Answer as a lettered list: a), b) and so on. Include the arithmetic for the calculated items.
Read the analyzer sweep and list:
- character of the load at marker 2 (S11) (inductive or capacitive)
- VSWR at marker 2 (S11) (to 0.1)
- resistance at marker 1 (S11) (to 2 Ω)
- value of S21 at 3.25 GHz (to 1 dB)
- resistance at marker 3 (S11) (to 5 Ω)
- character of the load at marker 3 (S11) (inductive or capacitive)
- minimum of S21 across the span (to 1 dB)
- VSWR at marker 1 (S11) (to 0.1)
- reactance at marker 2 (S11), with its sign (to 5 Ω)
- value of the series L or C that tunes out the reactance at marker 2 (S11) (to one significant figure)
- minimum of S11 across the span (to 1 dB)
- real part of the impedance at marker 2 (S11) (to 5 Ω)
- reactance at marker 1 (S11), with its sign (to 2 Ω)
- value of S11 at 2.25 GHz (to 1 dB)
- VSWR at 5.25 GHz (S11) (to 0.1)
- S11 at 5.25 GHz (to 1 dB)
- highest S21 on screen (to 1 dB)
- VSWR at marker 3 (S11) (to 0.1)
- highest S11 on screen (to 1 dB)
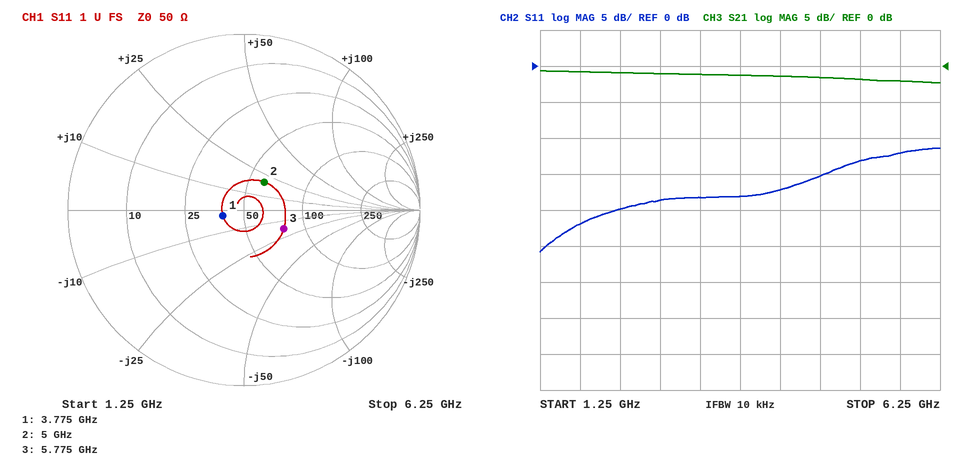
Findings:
a) inductive
b) 1.5
c) 40 Ω
d) -1 dB
e) 75 Ω
f) capacitive
g) -2 dB
h) 1.3
i) +20 Ω
j) C = 1/(2π × 5 GHz × 20 Ω) ≈ 2 pF
k) -26 dB
l) 60 Ω
m) -2 Ω
n) -20 dB
o) |Γ| = 10^(-13/20) = 0.2239; VSWR = (1 + 0.2239)/(1 − 0.2239) ≈ 1.6
p) -13 dB
q) -1 dB
r) 1.7
s) -11 dB
